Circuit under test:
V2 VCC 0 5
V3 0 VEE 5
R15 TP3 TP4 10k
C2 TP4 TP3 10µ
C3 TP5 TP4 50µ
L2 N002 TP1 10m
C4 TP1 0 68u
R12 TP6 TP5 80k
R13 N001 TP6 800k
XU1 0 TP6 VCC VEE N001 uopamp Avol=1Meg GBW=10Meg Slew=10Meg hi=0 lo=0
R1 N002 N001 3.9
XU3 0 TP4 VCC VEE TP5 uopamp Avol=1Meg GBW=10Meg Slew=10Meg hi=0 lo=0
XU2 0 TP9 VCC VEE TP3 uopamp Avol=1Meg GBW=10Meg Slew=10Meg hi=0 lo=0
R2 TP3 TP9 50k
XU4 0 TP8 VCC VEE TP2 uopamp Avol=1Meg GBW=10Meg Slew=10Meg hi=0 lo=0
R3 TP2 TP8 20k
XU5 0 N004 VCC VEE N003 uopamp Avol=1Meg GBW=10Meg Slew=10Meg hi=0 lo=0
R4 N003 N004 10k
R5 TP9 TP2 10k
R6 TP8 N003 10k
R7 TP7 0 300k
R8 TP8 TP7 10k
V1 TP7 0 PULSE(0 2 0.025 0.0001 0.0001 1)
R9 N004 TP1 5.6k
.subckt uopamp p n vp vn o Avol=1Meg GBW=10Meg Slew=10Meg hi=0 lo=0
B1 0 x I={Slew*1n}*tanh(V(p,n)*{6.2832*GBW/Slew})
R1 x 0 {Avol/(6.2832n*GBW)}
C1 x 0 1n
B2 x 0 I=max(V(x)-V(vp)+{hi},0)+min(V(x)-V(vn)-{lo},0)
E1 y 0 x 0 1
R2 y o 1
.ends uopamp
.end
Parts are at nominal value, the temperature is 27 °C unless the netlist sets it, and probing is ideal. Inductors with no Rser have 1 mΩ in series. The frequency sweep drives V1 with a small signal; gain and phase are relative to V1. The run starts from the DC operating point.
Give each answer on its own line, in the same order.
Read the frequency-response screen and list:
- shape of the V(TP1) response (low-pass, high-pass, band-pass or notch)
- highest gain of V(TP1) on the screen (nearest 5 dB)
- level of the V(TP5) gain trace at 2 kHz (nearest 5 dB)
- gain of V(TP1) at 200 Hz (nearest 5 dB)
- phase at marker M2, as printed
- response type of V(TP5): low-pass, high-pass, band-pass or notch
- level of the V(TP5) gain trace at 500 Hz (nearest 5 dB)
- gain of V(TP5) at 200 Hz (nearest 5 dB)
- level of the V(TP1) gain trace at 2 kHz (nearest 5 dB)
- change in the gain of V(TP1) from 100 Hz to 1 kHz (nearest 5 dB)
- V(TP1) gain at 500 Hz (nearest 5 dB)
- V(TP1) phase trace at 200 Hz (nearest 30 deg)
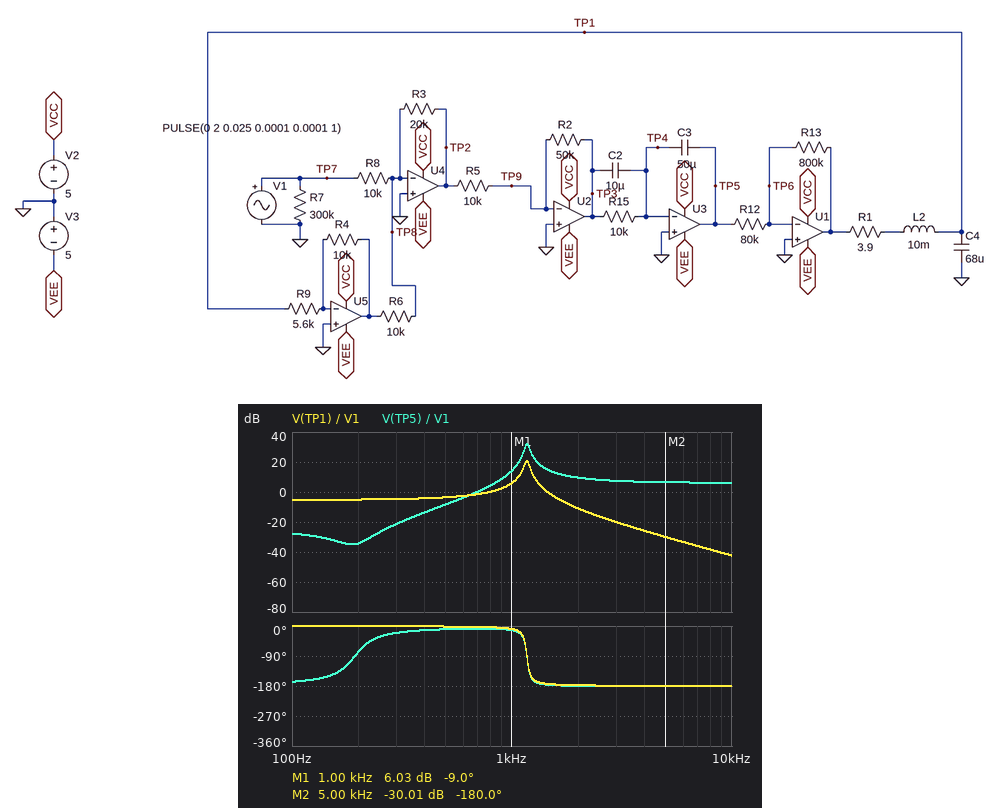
low-pass
20 dB
10 dB
-5 dB
-180.0 deg
band-pass
-10 dB
-35 dB
-10 dB
10 dB
-5 dB
0 deg
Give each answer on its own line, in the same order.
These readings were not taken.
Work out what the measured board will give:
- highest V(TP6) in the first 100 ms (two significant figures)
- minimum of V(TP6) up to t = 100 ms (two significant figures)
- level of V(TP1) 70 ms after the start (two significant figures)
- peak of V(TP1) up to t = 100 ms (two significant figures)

470 mV
-480 mV
1.1 V
1.7 V
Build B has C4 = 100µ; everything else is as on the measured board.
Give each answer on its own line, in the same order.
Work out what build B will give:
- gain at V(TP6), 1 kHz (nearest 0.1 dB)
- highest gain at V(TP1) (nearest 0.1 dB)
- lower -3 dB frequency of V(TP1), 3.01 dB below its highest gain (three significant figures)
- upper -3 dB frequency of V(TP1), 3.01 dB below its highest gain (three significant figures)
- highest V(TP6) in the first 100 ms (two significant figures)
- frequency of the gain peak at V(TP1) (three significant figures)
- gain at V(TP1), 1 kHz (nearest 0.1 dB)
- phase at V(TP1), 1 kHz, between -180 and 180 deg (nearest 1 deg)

-33.4 dB
19.1 dB
934 Hz
992 Hz
470 mV
963 Hz
14.9 dB
-140 deg
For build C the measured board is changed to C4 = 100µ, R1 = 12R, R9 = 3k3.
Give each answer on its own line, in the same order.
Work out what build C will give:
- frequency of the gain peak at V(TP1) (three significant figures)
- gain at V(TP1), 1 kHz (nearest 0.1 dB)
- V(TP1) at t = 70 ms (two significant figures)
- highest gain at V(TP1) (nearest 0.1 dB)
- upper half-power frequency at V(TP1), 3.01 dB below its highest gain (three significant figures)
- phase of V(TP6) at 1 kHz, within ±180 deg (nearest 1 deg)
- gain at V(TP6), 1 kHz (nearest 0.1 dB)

1.24 kHz
-1.3 dB
650 mV
6.8 dB
1.33 kHz
59 deg
-49.4 dB
